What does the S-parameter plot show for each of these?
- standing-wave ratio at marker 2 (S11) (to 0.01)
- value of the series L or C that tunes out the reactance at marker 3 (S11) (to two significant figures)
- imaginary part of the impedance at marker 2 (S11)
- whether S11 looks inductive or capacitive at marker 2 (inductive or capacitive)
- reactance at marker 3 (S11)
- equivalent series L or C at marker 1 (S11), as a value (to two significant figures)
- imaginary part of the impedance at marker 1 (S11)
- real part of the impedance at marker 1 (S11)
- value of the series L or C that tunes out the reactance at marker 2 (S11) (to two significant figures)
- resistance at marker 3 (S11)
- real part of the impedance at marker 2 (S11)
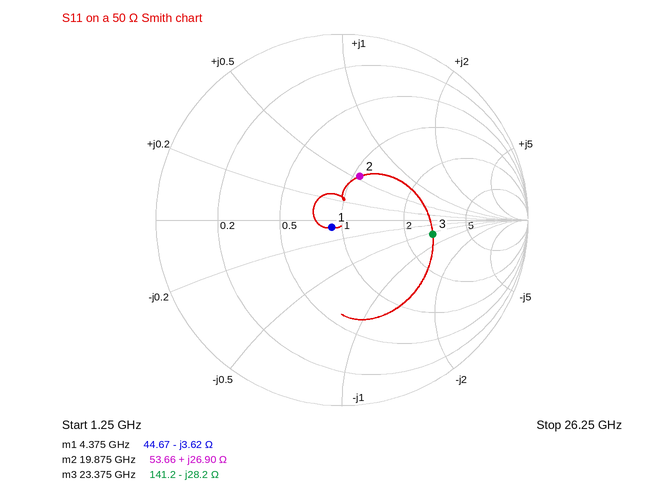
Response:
1.68
190 pH
+26.90 Ω
inductive
-28.2 Ω
10 pF
-3.62 Ω
44.67 Ω
300 fF
141.2 Ω
53.66 Ω
